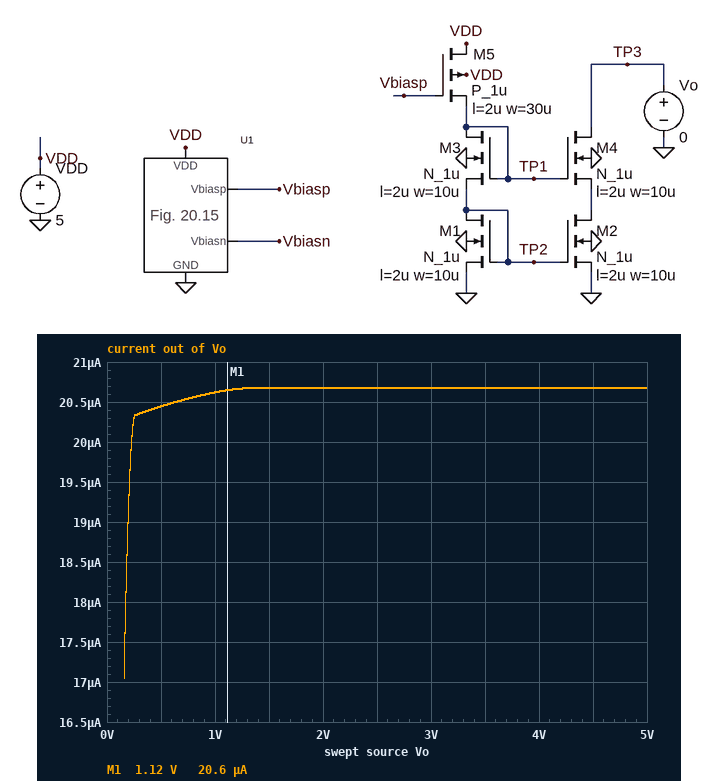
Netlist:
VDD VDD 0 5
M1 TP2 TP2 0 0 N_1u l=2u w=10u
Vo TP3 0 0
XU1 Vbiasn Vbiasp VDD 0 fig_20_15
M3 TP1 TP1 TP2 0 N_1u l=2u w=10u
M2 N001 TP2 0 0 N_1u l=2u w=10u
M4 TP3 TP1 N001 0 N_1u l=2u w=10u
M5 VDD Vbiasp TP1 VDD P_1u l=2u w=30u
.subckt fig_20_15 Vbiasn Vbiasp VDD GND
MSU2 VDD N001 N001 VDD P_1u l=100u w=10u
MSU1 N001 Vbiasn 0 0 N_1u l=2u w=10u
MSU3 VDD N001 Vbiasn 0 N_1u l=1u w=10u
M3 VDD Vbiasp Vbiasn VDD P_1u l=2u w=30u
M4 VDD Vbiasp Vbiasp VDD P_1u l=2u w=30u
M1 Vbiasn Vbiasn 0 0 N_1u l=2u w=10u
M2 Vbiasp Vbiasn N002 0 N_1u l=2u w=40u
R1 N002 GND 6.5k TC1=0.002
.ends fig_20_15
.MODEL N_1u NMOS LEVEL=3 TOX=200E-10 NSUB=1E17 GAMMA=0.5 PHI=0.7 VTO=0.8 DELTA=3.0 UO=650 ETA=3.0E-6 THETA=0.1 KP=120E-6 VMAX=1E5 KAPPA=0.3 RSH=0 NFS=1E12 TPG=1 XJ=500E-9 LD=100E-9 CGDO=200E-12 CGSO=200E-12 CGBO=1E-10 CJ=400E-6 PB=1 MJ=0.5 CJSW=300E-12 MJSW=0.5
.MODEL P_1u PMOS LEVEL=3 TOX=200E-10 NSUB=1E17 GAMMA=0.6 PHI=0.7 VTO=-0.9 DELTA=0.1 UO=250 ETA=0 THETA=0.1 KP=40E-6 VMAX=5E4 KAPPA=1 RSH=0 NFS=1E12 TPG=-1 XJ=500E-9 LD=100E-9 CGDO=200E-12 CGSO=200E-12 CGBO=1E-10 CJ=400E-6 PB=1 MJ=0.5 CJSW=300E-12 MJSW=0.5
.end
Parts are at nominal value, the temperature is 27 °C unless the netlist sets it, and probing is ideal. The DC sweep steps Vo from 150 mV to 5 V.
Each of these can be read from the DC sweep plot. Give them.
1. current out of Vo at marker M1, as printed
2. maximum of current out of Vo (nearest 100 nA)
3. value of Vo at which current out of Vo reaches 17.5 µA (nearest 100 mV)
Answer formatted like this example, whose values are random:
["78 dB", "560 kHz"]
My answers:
["20.6 µA", "20.7 µA", "200 mV"]
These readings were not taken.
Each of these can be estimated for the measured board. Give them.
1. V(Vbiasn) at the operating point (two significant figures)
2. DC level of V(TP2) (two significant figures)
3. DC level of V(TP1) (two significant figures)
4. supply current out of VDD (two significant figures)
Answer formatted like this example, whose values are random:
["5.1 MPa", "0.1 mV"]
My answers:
["1.1 V", "1.1 V", "2.4 V", "81 µA"]
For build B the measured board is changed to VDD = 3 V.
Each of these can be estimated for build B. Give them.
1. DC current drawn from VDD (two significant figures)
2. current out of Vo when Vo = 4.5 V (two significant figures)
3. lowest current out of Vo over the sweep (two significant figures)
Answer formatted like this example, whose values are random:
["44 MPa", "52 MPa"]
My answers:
["63 µA", "19 µA", "16 µA"]
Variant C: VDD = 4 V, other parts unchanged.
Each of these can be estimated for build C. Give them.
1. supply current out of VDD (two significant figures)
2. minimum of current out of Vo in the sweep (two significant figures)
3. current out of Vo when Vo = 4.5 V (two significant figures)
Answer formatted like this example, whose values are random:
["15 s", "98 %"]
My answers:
["71 µA", "16 µA", "20 µA"]
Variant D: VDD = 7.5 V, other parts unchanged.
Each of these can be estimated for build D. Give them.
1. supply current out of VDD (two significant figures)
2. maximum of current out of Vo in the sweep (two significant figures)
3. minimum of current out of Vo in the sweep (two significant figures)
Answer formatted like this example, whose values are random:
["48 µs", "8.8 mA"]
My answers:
["93 µA", "23 µA", "18 µA"]
